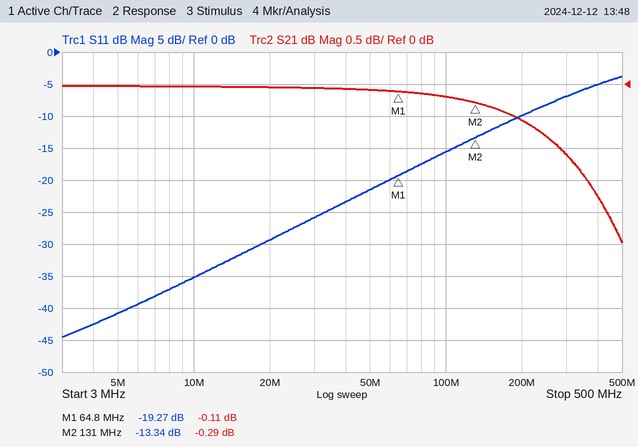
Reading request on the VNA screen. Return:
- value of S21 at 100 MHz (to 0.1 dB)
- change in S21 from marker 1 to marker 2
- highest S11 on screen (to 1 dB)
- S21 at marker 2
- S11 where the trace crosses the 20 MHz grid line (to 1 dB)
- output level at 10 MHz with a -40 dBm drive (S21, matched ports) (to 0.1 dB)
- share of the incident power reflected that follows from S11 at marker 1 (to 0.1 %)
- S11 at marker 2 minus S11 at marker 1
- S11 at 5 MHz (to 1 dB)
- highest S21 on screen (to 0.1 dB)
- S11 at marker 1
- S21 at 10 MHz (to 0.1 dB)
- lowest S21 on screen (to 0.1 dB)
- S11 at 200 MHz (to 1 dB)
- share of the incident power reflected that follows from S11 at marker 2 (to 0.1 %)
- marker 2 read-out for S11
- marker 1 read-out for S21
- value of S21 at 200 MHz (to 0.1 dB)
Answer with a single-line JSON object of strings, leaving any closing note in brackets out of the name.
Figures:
{"value of S21 at 100 MHz": "-0.2 dB", "change in S21 from marker 1 to marker 2": "-0.18 dB", "highest S11 on screen": "-4 dB", "S21 at marker 2": "-0.29 dB", "S11 where the trace crosses the 20 MHz grid line": "-29 dB", "output level at 10 MHz with a -40 dBm drive (S21, matched ports)": "-40.0 dBm", "share of the incident power reflected that follows from S11 at marker 1": "1.2 %", "S11 at marker 2 minus S11 at marker 1": "5.93 dB", "S11 at 5 MHz": "-41 dB", "highest S21 on screen": "0.0 dB", "S11 at marker 1": "-19.27 dB", "S21 at 10 MHz": "0.0 dB", "lowest S21 on screen": "-2.5 dB", "S11 at 200 MHz": "-10 dB", "share of the incident power reflected that follows from S11 at marker 2": "4.6 %", "marker 2 read-out for S11": "-13.34 dB", "marker 1 read-out for S21": "-0.11 dB", "value of S21 at 200 MHz": "-0.6 dB"}
